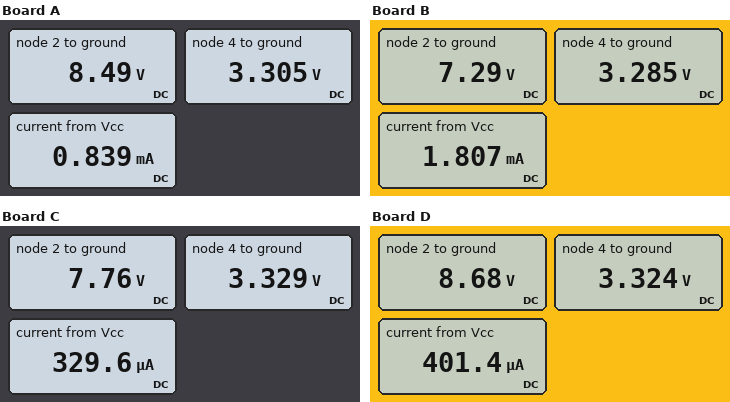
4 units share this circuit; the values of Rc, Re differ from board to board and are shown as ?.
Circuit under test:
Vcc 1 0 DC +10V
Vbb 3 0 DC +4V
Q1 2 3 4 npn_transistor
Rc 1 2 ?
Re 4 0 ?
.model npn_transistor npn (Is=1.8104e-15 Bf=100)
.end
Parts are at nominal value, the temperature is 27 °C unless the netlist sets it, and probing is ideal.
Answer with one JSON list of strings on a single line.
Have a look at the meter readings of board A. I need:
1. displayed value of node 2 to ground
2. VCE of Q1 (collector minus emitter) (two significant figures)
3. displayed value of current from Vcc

["8.49 V", "5.2 V", "0.839 mA"]
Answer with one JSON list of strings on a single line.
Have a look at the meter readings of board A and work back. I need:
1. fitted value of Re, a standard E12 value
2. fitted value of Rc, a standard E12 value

["3.9 kΩ", "1.8 kΩ"]
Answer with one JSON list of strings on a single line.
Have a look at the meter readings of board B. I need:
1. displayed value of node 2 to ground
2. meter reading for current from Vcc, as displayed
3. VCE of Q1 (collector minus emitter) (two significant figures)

["7.29 V", "1.807 mA", "4.0 V"]
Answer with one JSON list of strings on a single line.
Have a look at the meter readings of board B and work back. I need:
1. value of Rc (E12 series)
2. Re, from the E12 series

["1.5 kΩ", "1.8 kΩ"]
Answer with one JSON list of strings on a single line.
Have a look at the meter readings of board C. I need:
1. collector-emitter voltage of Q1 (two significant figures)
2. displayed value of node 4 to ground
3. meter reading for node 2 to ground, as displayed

["4.4 V", "3.329 V", "7.76 V"]
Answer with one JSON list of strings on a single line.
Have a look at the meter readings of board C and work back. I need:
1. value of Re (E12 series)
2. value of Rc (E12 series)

["10 kΩ", "6.8 kΩ"]
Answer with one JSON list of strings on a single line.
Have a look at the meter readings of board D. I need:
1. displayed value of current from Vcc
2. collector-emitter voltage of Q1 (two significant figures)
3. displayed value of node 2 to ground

["401.4 µA", "5.4 V", "8.68 V"]
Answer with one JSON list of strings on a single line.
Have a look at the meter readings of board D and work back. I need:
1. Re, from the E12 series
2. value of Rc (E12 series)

["8.2 kΩ", "3.3 kΩ"]
